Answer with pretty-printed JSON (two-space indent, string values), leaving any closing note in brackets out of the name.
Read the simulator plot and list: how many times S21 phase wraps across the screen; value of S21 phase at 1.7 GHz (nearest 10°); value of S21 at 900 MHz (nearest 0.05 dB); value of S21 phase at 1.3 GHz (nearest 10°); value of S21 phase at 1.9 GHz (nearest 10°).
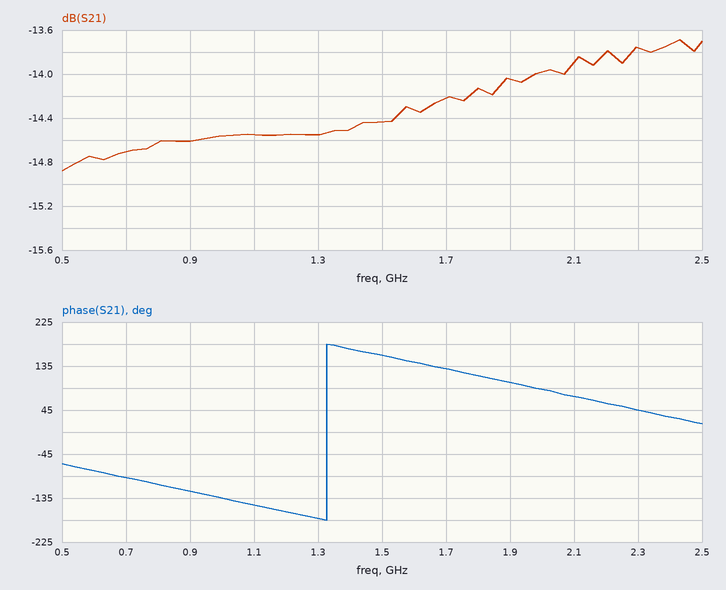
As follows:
{
  "how many times S21 phase wraps across the screen": "1",
  "value of S21 phase at 1.7 GHz": "130°",
  "value of S21 at 900 MHz": "-14.60 dB",
  "value of S21 phase at 1.3 GHz": "-180°",
  "value of S21 phase at 1.9 GHz": "100°"
}
